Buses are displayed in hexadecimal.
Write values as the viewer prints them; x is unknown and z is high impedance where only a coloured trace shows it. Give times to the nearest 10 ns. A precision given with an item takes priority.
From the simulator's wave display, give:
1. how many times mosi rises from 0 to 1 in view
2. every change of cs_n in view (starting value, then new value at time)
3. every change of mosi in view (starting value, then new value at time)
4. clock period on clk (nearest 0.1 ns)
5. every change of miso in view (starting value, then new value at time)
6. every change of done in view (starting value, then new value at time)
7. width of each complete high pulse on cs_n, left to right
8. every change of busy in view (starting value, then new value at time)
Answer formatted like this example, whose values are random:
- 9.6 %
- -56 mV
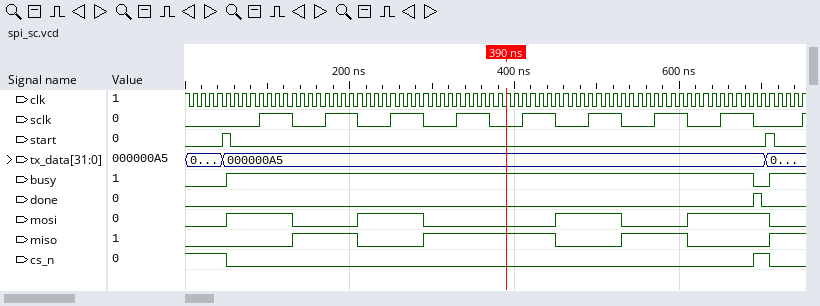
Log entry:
- 4
- 1, 0 at 50 ns, 1 at 690 ns, 0 at 710 ns
- 0, 1 at 50 ns, 0 at 130 ns, 1 at 210 ns, 0 at 290 ns, 1 at 450 ns, 0 at 530 ns, 1 at 610 ns, 0 at 710 ns
- 10 ns
- 0, 1 at 130 ns, 0 at 210 ns, 1 at 290 ns, 0 at 450 ns, 1 at 530 ns, 0 at 610 ns, 1 at 710 ns
- 0, 1 at 690 ns, 0 at 700 ns
- 20 ns
- 0, 1 at 50 ns, 0 at 690 ns, 1 at 710 ns
